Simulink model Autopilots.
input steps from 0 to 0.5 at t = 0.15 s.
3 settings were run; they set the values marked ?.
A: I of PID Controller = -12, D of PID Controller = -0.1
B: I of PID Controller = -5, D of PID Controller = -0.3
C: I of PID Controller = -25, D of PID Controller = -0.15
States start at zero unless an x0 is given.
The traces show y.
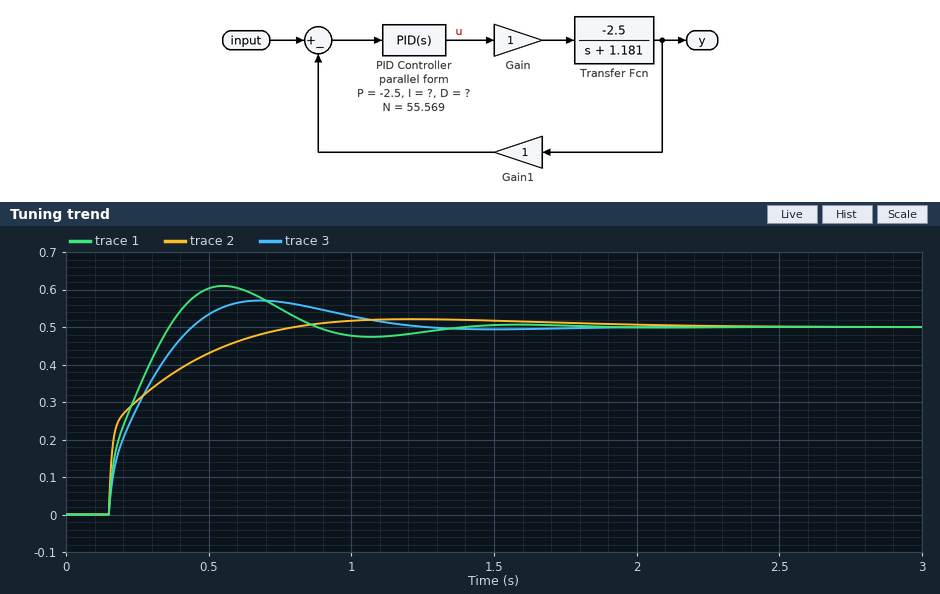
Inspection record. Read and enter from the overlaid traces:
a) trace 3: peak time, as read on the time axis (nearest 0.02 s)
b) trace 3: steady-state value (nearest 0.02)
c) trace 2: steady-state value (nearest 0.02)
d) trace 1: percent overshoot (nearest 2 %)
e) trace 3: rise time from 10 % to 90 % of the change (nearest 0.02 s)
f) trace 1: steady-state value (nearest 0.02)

0.68 s
0.50
0.50
22 %
0.22 s
0.50
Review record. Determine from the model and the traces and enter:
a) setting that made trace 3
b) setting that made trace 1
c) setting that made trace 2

A
C
B
